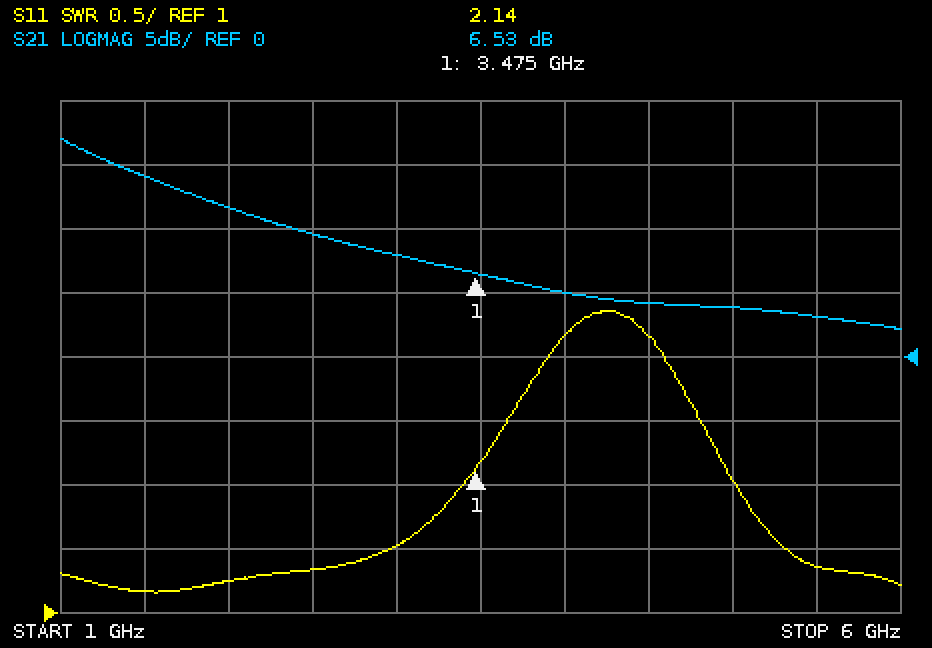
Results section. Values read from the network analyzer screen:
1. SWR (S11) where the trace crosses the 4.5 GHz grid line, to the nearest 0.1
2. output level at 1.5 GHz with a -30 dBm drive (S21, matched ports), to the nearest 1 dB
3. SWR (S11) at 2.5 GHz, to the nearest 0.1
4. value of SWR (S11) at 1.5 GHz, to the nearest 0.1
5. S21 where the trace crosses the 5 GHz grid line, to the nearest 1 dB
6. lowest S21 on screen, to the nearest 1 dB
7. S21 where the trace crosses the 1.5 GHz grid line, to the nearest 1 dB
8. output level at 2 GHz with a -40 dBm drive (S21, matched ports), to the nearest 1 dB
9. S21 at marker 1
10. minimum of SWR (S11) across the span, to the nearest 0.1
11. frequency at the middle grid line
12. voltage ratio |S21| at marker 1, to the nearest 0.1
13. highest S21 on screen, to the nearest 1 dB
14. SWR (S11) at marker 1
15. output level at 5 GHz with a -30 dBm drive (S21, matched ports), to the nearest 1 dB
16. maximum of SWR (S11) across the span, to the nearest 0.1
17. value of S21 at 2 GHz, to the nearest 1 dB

3.2
-16 dBm
1.3
1.2
4 dB
2 dB
14 dB
-28 dBm
6.53 dB
1.2
3.5 GHz
2.1
17 dB
2.14
-26 dBm
3.4
12 dB
